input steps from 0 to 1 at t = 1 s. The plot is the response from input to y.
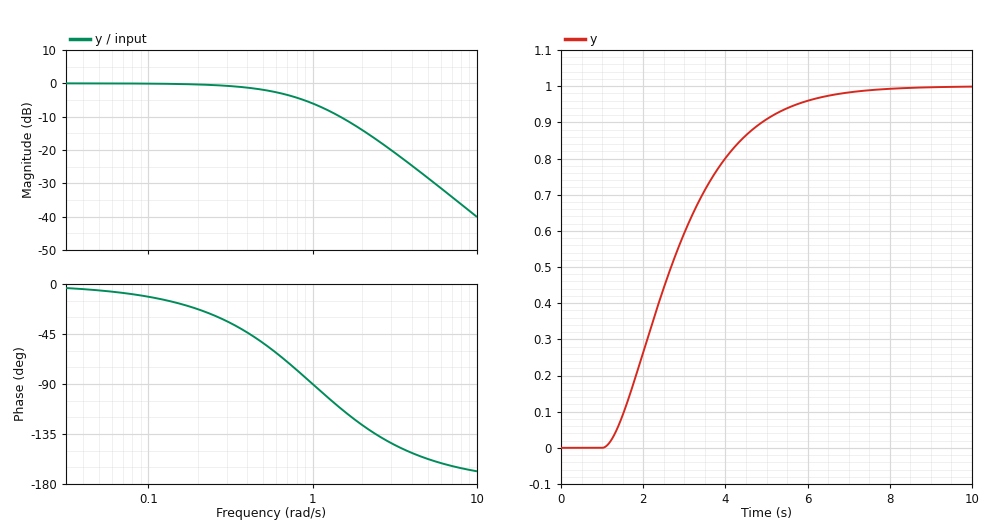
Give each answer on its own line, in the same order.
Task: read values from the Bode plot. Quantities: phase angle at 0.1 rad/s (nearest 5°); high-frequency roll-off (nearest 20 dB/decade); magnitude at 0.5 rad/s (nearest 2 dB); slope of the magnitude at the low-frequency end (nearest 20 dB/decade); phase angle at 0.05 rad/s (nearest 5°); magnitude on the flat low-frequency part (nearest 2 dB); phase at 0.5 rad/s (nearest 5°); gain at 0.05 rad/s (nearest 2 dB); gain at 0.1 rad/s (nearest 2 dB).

-10°
-40 dB/decade
-2 dB
0 dB/decade
-5°
0 dB
-55°
0 dB
0 dB
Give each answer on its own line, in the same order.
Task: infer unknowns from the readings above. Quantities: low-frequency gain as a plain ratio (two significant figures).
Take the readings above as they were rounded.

1.0
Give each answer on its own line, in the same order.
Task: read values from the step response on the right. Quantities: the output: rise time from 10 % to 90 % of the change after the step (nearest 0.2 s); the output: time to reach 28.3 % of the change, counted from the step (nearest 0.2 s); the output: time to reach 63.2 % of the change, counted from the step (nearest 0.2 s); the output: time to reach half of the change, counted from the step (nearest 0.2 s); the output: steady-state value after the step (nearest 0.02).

3.4 s
1.0 s
2.2 s
1.6 s
1.00
